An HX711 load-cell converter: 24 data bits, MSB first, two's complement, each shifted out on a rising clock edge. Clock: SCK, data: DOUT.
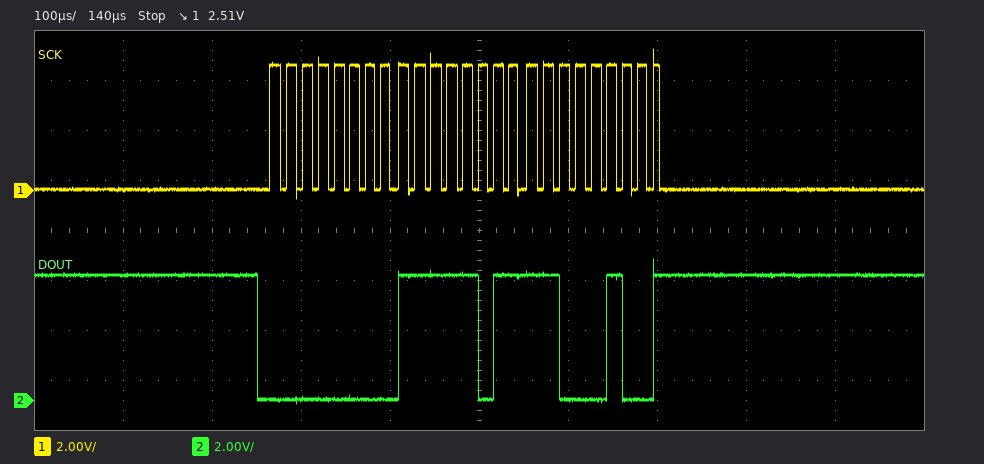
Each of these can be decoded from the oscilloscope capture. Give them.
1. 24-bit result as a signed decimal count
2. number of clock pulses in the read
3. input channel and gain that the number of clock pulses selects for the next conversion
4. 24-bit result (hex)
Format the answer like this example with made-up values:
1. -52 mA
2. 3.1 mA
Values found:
1. 64452
2. 25
3. channel A, gain 128
4. 0x00FBC4
